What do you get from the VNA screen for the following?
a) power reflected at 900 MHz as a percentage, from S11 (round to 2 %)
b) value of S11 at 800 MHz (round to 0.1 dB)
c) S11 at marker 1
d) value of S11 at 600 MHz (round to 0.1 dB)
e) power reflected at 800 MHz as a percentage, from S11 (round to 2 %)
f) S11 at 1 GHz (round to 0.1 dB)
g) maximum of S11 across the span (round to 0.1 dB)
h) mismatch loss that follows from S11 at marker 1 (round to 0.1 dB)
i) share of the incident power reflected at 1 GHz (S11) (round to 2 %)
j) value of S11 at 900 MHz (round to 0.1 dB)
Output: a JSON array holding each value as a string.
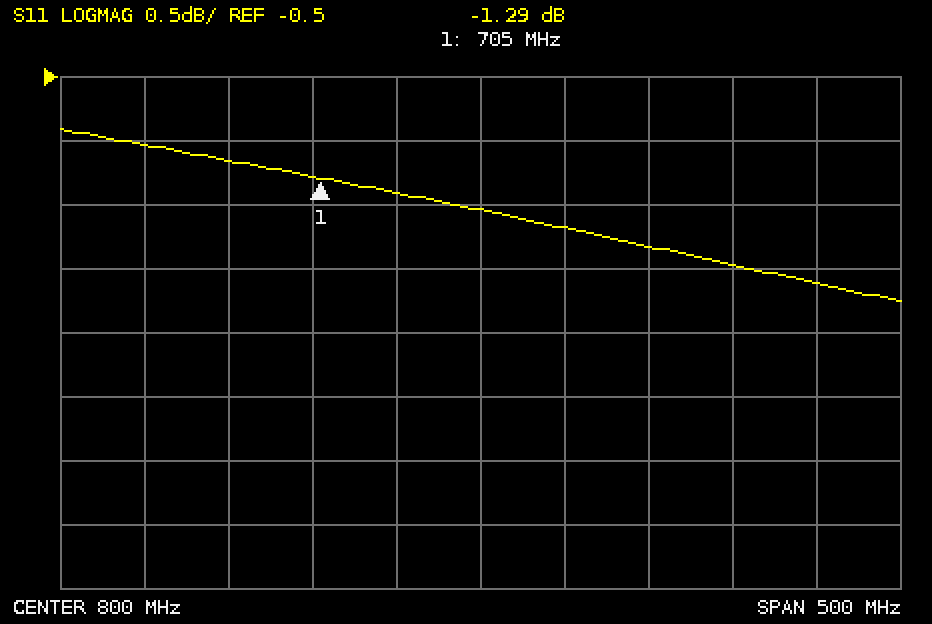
["66 %", "-1.5 dB", "-1.29 dB", "-1.0 dB", "70 %", "-2.1 dB", "-0.9 dB", "5.9 dB", "62 %", "-1.8 dB"]
